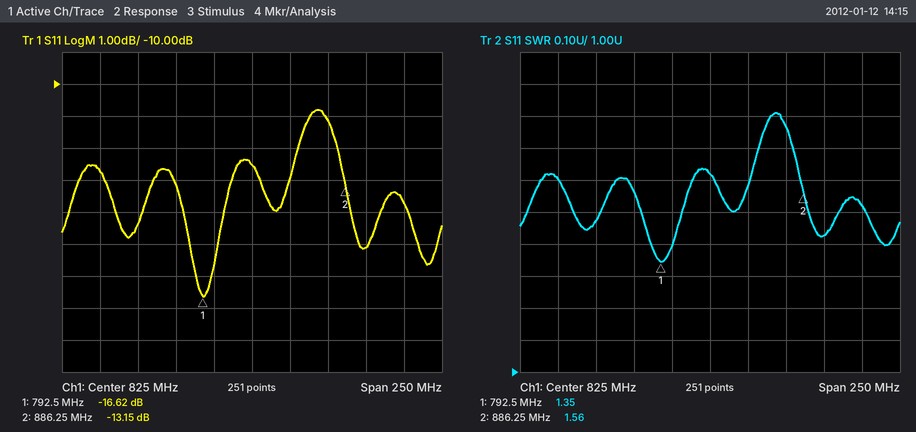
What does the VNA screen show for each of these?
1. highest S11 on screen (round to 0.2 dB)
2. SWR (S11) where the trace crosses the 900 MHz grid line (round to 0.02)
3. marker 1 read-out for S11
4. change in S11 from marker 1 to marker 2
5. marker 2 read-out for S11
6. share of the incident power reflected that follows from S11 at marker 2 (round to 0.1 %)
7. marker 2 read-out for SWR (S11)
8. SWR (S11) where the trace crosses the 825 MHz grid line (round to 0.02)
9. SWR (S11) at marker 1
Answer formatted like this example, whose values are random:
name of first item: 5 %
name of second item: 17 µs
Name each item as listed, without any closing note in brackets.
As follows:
highest S11 on screen: -10.8 dB
SWR (S11) where the trace crosses the 900 MHz grid line: 1.42
marker 1 read-out for S11: -16.62 dB
change in S11 from marker 1 to marker 2: 3.47 dB
marker 2 read-out for S11: -13.15 dB
share of the incident power reflected that follows from S11 at marker 2: 4.8 %
marker 2 read-out for SWR: 1.56
SWR (S11) where the trace crosses the 825 MHz grid line: 1.62
SWR (S11) at marker 1: 1.35
